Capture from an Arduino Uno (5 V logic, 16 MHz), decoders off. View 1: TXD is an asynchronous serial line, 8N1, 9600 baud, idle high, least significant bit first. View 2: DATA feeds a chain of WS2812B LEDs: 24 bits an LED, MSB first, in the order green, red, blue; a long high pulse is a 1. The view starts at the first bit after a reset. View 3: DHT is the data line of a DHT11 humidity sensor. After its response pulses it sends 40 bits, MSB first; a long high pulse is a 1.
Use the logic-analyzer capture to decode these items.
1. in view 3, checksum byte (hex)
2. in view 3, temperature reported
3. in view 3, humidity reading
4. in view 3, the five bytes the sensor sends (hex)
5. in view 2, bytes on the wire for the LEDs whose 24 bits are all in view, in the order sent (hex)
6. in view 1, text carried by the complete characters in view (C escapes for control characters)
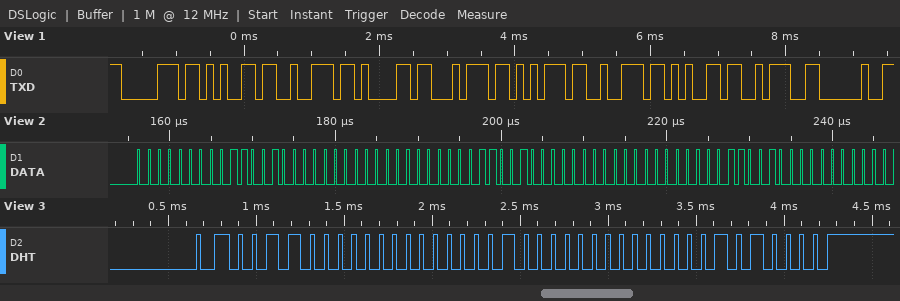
0x50
32.0 °C
48 %
30 00 20 00 50
00 64 00 00 64 00 00 64 00
"perature: "
